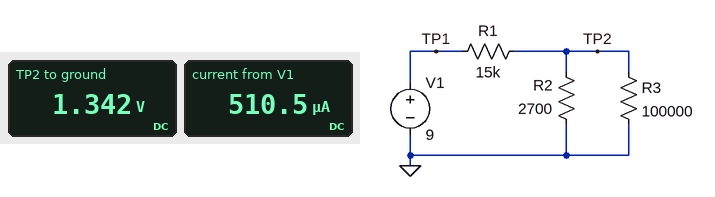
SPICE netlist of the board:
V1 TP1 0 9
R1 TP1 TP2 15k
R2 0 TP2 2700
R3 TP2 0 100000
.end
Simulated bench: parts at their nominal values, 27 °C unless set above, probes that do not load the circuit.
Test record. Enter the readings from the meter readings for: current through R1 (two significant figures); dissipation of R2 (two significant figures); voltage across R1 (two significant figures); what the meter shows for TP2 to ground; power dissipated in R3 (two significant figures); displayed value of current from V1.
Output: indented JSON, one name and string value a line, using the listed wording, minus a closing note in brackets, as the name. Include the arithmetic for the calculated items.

{
  "current through R1": "(9 V - 1.342 V) / 15 kΩ = 510 µA",
  "dissipation of R2": "(1.342 V)^2 / 2.7 kΩ = 670 µW",
  "voltage across R1": "9 V - 1.342 V = 7.7 V",
  "what the meter shows for TP2 to ground": "1.342 V",
  "power dissipated in R3": "(1.342 V)^2 / 100 kΩ = 18 µW",
  "displayed value of current from V1": "510.5 µA"
}
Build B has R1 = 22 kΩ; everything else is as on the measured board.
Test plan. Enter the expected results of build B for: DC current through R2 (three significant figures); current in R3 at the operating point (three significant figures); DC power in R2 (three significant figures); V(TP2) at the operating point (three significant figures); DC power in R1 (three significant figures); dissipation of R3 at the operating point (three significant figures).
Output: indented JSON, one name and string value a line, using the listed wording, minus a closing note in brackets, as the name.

{
  "DC current through R2": "356 µA",
  "current in R3 at the operating point": "9.61 µA",
  "DC power in R2": "342 µW",
  "V(TP2) at the operating point": "961 mV",
  "DC power in R1": "2.94 mW",
  "dissipation of R3 at the operating point": "9.23 µW"
}
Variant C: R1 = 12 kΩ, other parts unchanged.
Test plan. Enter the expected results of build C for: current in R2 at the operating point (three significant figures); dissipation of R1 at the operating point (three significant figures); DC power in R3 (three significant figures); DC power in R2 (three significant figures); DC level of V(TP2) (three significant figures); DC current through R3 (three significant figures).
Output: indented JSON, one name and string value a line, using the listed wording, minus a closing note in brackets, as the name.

{
  "current in R2 at the operating point": "599 µA",
  "dissipation of R1 at the operating point": "4.54 mW",
  "DC power in R3": "26.2 µW",
  "DC power in R2": "969 µW",
  "DC level of V(TP2)": "1.62 V",
  "DC current through R3": "16.2 µA"
}
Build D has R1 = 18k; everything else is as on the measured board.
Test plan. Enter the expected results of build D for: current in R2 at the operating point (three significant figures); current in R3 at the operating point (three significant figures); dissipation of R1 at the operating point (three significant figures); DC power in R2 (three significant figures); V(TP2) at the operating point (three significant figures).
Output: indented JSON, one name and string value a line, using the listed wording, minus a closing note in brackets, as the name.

{
  "current in R2 at the operating point": "425 µA",
  "current in R3 at the operating point": "11.5 µA",
  "dissipation of R1 at the operating point": "3.43 mW",
  "DC power in R2": "487 µW",
  "V(TP2) at the operating point": "1.15 V"
}
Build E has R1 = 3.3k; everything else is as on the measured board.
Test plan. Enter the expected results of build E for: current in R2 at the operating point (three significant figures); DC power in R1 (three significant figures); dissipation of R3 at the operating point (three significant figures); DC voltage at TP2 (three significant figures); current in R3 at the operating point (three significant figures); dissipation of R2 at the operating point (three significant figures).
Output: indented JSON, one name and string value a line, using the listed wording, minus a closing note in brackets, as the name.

{
  "current in R2 at the operating point": "1.48 mA",
  "DC power in R1": "7.60 mW",
  "dissipation of R3 at the operating point": "159 µW",
  "DC voltage at TP2": "3.99 V",
  "current in R3 at the operating point": "39.9 µA",
  "dissipation of R2 at the operating point": "5.90 mW"
}
